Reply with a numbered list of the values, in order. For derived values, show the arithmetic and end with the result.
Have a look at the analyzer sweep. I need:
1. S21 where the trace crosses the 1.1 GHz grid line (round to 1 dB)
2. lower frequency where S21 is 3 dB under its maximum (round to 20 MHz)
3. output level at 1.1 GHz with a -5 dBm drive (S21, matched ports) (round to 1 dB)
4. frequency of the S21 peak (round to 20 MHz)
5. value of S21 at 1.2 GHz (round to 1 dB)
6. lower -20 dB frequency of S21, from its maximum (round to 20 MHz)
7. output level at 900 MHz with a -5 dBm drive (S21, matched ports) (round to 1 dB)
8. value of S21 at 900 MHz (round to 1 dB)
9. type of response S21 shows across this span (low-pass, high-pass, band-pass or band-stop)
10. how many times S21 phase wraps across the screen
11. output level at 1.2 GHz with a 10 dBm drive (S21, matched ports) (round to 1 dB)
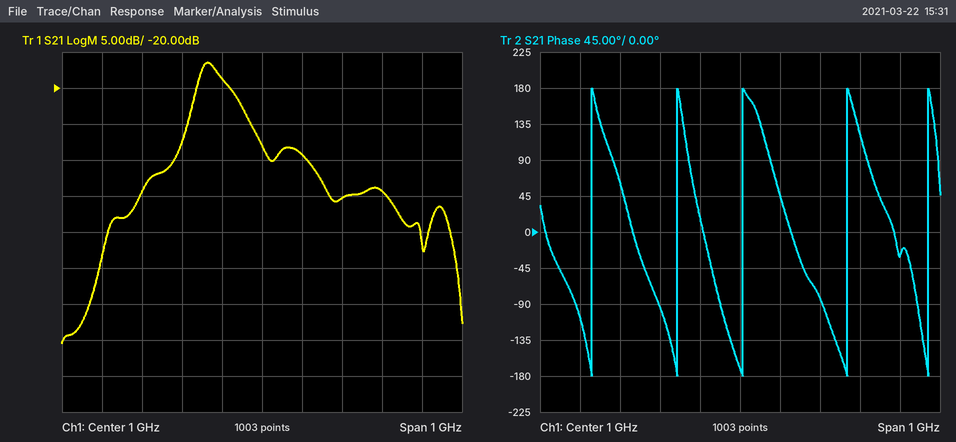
1. -29 dB
2. 840 MHz
3. -5 dBm + (-29 dB) = -34 dBm
4. 860 MHz
5. -35 dB
6. 680 MHz
7. -5 dBm + (-19 dB) = -24 dBm
8. -19 dB
9. band-pass
10. 5
11. 10 dBm + (-35 dB) = -25 dBm
